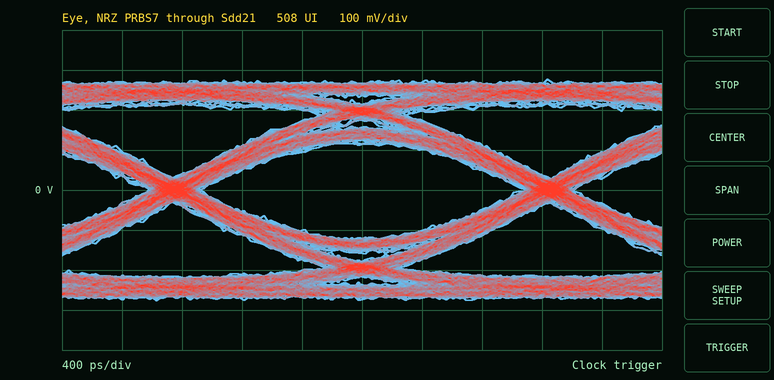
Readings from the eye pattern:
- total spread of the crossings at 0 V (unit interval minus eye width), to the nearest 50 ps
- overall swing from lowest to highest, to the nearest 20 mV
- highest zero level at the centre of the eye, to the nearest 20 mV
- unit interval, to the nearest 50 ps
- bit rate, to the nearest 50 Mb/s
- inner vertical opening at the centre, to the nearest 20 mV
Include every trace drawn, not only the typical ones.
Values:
350 ps
560 mV
-120 mV
2.50 ns
400 Mb/s
240 mV
